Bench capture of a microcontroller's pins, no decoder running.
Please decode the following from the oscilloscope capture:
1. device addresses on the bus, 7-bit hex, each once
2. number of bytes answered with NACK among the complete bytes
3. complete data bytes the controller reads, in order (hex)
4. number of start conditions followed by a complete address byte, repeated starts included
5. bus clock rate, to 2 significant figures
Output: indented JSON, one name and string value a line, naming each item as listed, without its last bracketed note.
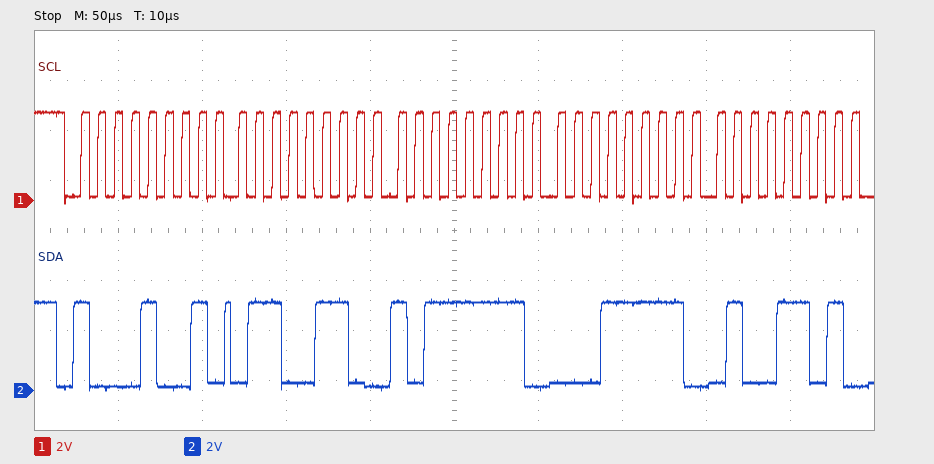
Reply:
{
  "device addresses on the bus, 7-bit hex, each once": "0x44",
  "number of bytes answered with NACK among the complete bytes": "0",
  "complete data bytes the controller reads, in order": "66 BF 1F 4D",
  "number of start conditions followed by a complete address byte, repeated starts included": "1",
  "bus clock rate, to 2 significant figures": "100 kHz"
}
